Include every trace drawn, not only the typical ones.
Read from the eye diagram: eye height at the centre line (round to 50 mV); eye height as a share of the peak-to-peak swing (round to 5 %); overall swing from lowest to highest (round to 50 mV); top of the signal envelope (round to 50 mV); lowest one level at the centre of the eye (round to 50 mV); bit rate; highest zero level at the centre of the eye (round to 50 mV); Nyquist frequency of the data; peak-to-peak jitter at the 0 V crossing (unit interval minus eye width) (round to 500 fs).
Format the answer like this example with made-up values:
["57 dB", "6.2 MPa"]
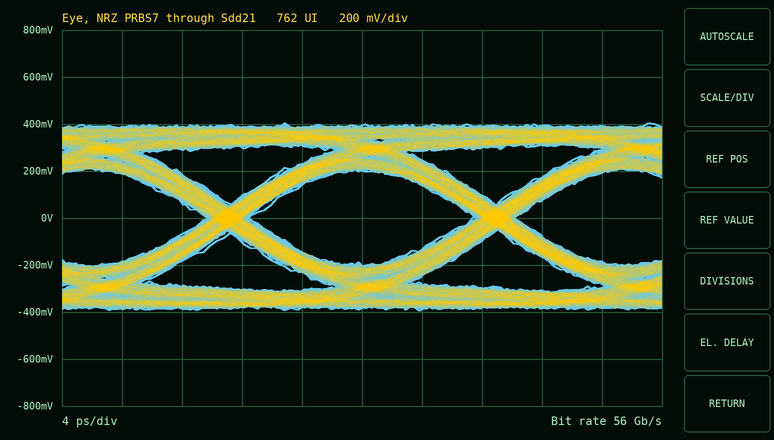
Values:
["400 mV", "50 %", "800 mV", "400 mV", "200 mV", "56 Gb/s", "-200 mV", "28 GHz", "3.0 ps"]
